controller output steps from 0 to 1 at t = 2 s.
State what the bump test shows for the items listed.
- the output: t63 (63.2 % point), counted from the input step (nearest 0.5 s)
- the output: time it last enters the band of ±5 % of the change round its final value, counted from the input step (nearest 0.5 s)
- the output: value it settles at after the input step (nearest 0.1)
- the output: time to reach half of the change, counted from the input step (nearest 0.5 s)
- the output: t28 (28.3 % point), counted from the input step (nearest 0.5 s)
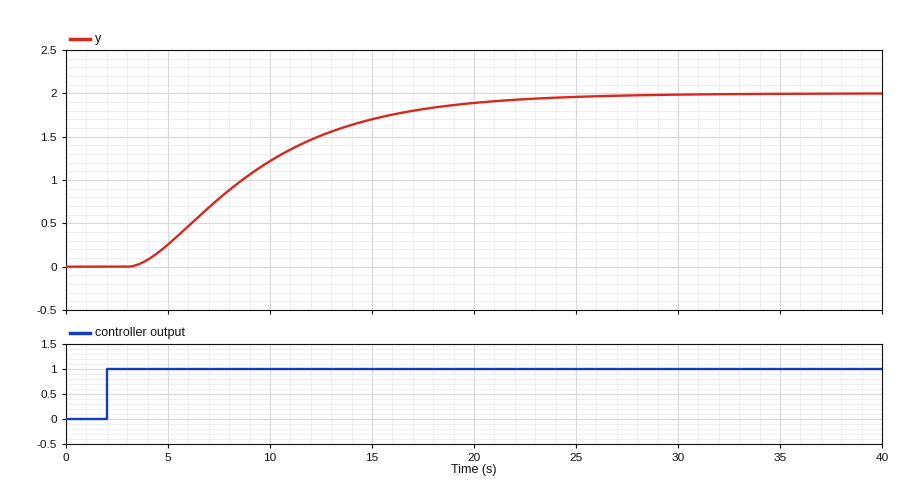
8.5 s
18.5 s
2.0
6.5 s
4.5 s
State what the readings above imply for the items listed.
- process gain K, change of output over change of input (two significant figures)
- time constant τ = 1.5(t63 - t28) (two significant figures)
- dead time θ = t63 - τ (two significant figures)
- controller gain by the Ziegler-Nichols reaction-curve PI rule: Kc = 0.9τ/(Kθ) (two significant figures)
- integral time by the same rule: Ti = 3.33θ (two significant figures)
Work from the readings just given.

2.0
6.0 s
2.5 s
1.1
8.3 s
